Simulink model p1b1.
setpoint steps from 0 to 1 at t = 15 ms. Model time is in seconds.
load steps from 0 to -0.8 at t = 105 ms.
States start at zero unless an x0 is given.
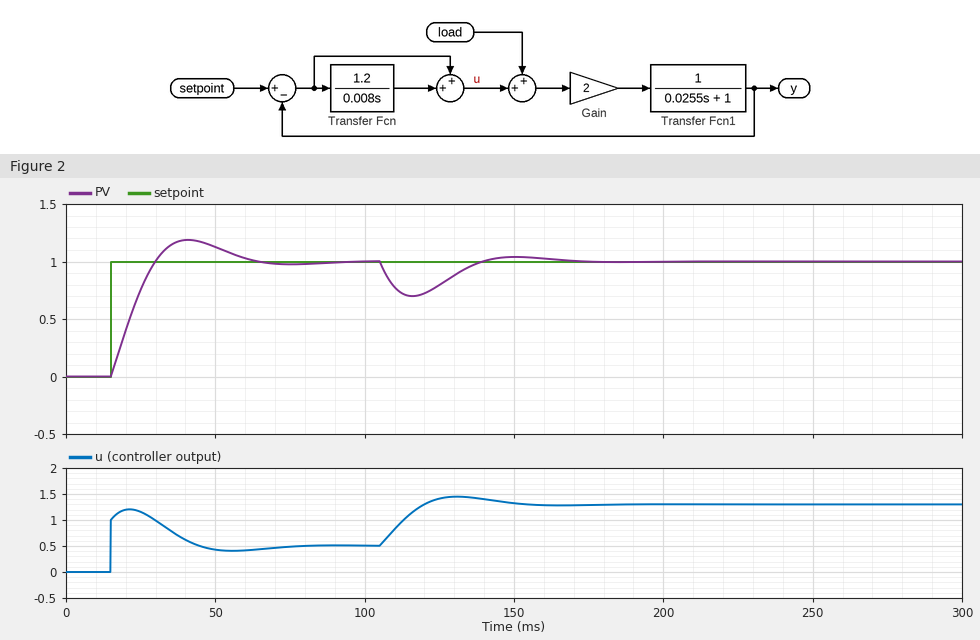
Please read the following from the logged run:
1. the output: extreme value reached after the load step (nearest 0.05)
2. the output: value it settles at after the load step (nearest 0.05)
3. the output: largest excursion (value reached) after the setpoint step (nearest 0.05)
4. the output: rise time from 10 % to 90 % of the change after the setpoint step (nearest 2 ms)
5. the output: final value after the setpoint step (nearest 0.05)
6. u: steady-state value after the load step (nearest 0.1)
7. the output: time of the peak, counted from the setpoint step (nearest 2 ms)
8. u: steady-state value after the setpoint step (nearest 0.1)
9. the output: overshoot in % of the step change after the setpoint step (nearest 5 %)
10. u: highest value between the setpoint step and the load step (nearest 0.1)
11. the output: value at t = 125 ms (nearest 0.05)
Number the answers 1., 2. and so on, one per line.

1. 0.70
2. 1.00
3. 1.20
4. 12 ms
5. 1.00
6. 1.3
7. 26 ms
8. 0.5
9. 20 %
10. 1.2
11. 0.80
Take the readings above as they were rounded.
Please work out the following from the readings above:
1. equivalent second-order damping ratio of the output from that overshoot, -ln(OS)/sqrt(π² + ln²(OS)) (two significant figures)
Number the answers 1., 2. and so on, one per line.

1. 0.46
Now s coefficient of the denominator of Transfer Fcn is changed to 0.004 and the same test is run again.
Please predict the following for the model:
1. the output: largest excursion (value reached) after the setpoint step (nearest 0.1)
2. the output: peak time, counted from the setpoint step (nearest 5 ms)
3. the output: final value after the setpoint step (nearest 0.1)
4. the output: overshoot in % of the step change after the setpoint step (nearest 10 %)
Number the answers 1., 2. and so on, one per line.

1. 1.3
2. 20 ms
3. 1.0
4. 30 %
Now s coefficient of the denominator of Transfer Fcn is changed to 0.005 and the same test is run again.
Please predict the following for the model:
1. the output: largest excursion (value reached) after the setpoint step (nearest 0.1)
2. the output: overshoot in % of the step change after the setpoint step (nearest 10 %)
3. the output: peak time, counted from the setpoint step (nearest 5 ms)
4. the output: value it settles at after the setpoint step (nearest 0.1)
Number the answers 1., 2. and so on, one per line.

1. 1.3
2. 30 %
3. 20 ms
4. 1.0
